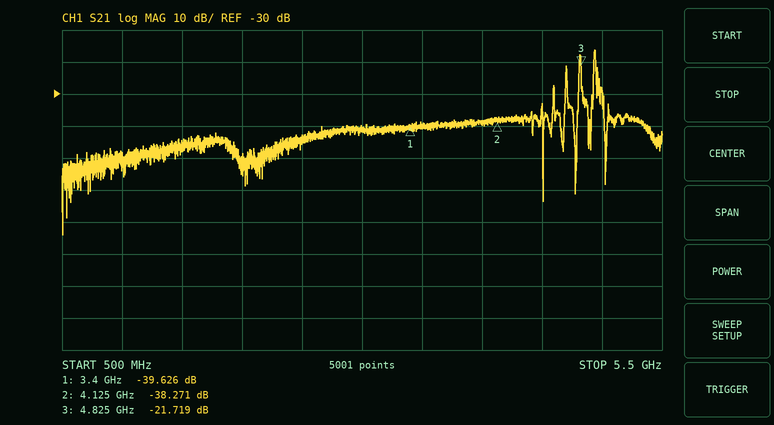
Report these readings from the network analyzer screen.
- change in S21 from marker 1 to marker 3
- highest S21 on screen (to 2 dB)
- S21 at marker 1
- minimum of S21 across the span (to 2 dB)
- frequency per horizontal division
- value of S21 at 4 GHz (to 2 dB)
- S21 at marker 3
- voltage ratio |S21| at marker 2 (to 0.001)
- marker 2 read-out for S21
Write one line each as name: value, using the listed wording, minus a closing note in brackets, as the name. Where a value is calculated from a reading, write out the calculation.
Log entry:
change in S21 from marker 1 to marker 3: -21.719 − (-39.626) = 17.907 dB
highest S21 on screen: -16 dB
S21 at marker 1: -39.626 dB
minimum of S21 across the span: -74 dB
frequency per horizontal division: 500 MHz
value of S21 at 4 GHz: -38 dB
S21 at marker 3: -21.719 dB
voltage ratio |S21| at marker 2: 10^(-38.271/20) ≈ 0.012
marker 2 read-out for S21: -38.271 dB
